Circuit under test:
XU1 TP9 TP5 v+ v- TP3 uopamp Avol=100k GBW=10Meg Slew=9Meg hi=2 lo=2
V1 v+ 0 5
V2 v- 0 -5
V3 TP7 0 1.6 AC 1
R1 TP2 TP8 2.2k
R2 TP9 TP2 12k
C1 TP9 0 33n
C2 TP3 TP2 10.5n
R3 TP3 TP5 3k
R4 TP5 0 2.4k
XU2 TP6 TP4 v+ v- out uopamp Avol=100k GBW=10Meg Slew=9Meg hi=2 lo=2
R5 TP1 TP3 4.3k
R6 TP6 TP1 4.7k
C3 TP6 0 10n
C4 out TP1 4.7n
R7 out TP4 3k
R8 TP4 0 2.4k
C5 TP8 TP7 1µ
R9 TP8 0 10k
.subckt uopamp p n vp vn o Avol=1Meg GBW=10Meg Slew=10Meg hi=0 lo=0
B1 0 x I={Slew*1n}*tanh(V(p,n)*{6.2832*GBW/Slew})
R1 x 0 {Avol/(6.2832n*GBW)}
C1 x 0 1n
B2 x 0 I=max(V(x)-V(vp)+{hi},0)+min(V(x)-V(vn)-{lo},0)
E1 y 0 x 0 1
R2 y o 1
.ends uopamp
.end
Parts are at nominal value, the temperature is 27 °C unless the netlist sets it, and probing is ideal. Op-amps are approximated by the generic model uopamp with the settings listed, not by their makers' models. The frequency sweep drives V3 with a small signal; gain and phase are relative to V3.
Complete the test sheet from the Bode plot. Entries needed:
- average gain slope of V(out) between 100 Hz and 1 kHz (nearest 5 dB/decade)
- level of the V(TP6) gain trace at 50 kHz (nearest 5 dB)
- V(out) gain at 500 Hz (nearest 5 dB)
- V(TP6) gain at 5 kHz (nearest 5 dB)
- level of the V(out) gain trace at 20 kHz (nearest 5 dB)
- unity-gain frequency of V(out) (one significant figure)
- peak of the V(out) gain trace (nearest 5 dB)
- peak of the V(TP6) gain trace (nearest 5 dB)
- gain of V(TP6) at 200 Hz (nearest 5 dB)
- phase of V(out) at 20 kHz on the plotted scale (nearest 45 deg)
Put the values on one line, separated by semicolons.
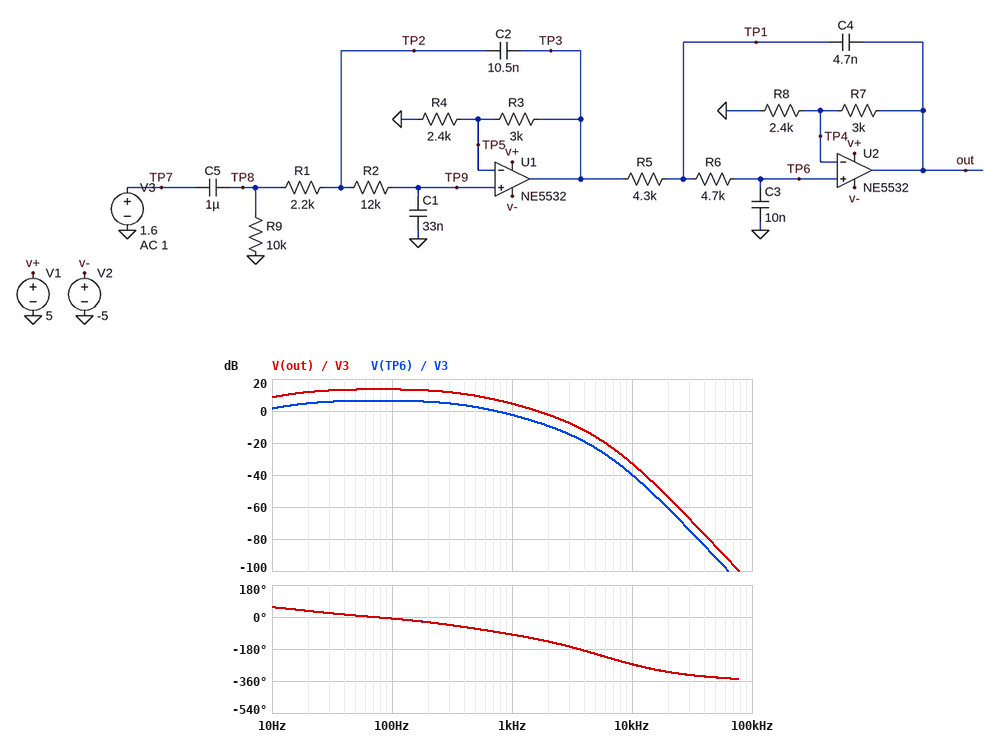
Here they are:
-10 dB/decade; -90 dB; 10 dB; -25 dB; -55 dB; 2 kHz; 15 dB; 5 dB; 5 dB; -315 deg
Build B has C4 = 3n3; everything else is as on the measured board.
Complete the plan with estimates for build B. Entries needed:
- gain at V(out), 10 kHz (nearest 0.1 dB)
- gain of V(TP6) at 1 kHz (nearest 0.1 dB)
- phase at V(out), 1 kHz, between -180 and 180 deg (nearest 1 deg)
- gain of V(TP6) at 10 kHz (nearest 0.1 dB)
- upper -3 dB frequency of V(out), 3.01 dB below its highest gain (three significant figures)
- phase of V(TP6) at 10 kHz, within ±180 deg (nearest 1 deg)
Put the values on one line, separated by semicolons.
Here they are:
-32.6 dB; -2.7 dB; -101 deg; -39.7 dB; 405 Hz; 109 deg
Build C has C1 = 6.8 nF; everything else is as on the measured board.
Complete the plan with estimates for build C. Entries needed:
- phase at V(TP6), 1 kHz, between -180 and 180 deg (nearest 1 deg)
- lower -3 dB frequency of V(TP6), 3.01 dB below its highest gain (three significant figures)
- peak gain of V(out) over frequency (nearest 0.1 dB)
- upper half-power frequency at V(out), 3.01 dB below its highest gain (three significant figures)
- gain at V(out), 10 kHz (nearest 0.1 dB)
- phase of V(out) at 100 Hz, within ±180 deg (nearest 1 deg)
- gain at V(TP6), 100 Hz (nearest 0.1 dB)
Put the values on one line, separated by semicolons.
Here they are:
-47 deg; 15.8 Hz; 14.1 dB; 2.27 kHz; -17.5 dB; 4 deg; 7.0 dB
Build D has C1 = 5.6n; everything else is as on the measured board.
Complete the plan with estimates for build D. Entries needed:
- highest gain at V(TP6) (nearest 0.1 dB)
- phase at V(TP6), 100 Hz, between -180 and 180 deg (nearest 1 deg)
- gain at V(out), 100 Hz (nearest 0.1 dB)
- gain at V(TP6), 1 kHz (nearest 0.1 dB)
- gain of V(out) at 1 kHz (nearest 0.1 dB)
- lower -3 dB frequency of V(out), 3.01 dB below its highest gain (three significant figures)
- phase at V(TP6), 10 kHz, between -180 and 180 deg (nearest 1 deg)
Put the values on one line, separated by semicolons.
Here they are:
7.1 dB; 5 deg; 14.0 dB; 6.8 dB; 13.8 dB; 15.9 Hz; 88 deg
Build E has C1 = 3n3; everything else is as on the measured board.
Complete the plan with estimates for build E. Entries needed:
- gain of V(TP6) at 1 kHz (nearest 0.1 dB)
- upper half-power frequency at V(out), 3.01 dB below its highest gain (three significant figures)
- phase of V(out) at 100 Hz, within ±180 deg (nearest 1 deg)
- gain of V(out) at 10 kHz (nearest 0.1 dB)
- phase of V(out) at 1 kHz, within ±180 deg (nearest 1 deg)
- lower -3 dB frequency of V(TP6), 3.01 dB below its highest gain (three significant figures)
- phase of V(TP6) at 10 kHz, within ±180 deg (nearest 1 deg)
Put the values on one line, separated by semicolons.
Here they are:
7.0 dB; 5.44 kHz; 6 deg; -8.9 dB; -29 deg; 16.0 Hz; 80 deg
